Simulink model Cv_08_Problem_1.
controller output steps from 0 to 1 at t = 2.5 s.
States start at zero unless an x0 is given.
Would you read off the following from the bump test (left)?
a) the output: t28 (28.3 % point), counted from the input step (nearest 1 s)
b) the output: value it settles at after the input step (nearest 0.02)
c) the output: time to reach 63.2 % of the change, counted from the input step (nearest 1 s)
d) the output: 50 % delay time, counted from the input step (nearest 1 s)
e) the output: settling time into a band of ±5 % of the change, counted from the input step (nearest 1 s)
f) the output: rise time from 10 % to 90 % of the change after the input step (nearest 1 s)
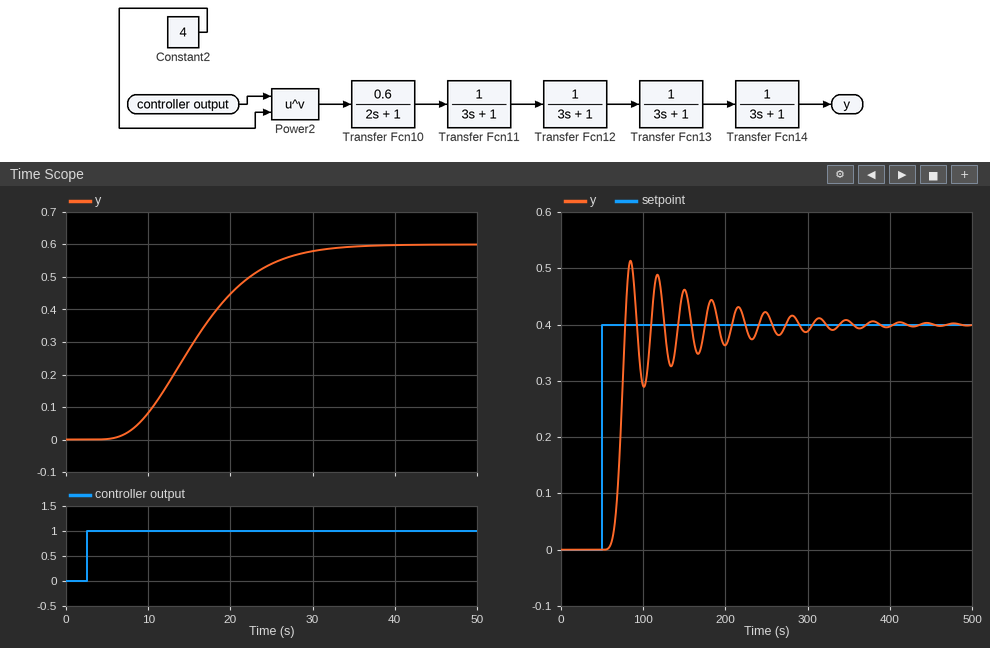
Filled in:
10 s
0.60
15 s
13 s
26 s
16 s
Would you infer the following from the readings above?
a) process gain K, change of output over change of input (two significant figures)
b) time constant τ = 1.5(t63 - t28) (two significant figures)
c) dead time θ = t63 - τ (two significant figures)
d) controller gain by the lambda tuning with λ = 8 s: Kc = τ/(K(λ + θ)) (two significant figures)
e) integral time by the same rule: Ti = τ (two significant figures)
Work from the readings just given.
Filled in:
0.60
7.5 s
7.5 s
0.81
7.5 s
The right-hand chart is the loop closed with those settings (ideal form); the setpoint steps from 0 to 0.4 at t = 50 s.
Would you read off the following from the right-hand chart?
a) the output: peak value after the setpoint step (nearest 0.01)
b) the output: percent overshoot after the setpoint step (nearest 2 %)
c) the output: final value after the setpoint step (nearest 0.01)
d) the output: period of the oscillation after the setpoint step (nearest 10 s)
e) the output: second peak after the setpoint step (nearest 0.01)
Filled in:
0.51
28 %
0.40
30 s
0.49
